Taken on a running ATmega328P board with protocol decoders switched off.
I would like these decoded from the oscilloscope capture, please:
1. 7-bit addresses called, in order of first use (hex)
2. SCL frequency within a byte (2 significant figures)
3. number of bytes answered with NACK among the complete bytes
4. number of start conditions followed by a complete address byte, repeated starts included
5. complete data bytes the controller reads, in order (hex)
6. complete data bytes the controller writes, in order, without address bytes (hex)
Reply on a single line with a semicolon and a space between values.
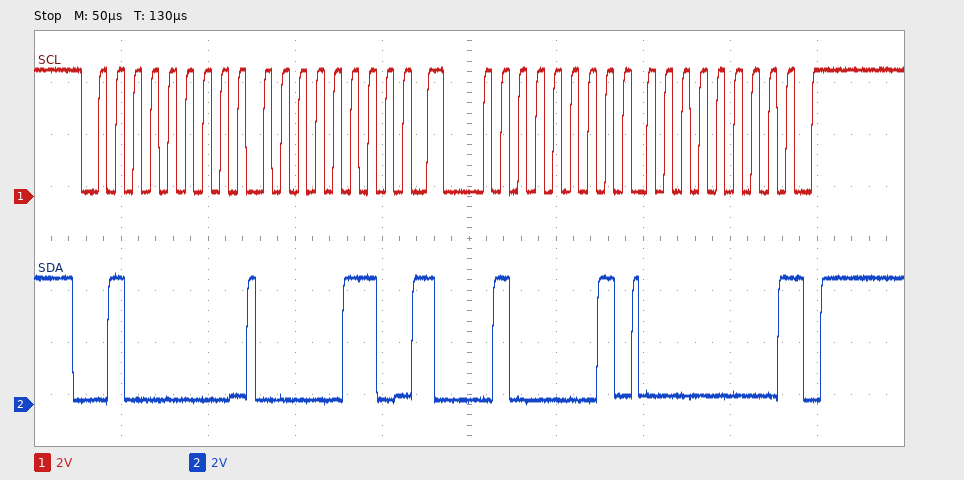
0x20; 100 kHz; 1; 2; 00; 06
